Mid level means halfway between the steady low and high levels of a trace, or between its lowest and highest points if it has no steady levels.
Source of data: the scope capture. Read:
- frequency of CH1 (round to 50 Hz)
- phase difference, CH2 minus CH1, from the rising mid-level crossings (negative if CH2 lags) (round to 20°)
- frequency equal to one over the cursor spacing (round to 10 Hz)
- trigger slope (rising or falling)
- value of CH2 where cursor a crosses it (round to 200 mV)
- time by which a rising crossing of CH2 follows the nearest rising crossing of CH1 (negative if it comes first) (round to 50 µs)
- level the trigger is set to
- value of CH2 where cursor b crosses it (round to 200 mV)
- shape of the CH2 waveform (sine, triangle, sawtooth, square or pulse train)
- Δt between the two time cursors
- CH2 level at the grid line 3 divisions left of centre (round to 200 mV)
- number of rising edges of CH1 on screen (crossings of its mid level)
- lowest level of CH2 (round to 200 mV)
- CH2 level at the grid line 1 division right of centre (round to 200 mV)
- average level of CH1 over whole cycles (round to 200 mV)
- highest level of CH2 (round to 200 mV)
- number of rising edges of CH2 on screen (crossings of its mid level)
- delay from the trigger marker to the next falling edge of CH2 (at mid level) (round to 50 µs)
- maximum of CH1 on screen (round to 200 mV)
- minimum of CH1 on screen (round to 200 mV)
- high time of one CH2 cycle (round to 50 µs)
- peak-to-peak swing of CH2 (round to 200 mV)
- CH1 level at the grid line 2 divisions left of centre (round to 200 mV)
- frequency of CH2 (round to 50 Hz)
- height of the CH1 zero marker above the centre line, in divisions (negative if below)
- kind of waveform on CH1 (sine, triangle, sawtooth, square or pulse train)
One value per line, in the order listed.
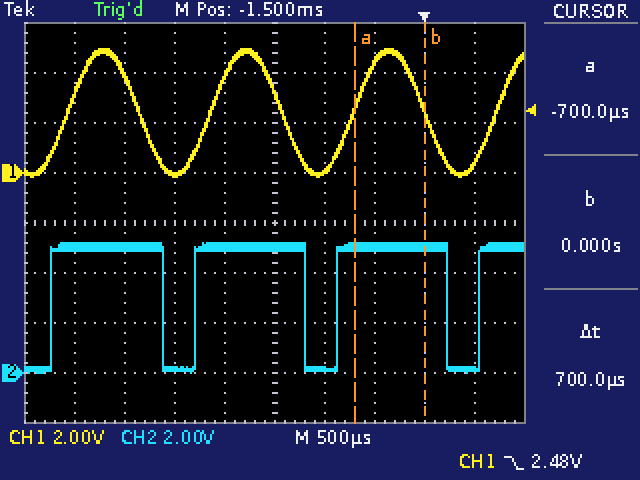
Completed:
700 Hz
+40°
1.43 kHz
falling
5.0 V
-150 µs
2.48 V
5.0 V
pulse train
700 µs
5.0 V
4
0.0 V
200 mV
2.4 V
5.2 V
4
250 µs
5.0 V
-200 mV
1.10 ms
5.2 V
0.0 V
700 Hz
+1.0 div
sine
